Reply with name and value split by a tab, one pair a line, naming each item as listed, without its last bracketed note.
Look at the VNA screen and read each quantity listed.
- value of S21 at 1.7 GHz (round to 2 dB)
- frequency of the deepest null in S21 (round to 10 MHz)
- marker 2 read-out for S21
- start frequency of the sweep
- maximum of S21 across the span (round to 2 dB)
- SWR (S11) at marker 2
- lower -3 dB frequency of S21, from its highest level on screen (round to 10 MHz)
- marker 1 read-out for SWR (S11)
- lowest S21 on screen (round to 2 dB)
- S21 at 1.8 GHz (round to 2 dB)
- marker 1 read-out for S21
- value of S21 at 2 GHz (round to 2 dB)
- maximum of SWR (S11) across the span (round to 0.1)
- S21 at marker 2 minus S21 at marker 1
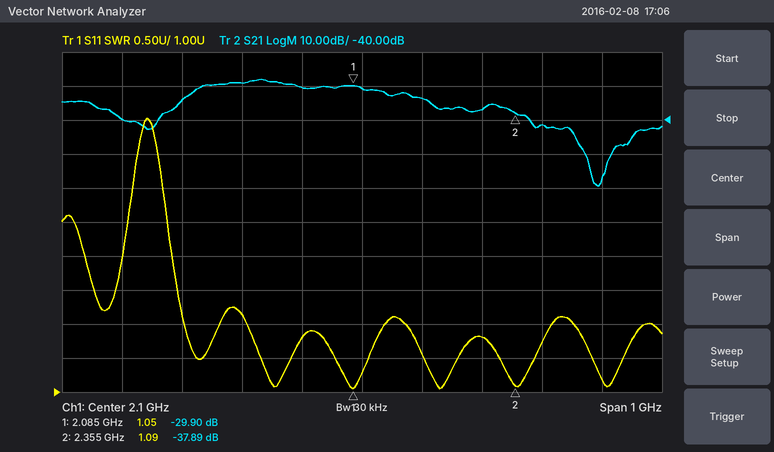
value of S21 at 1.7 GHz	-40 dB
frequency of the deepest null in S21	2.49 GHz
marker 2 read-out for S21	-37.89 dB
start frequency of the sweep	1.6 GHz
maximum of S21 across the span	-28 dB
SWR (S11) at marker 2	1.09
lower -3 dB frequency of S21, from its highest level on screen	1.82 GHz
marker 1 read-out for SWR	1.05
lowest S21 on screen	-60 dB
S21 at 1.8 GHz	-34 dB
marker 1 read-out for S21	-29.90 dB
value of S21 at 2 GHz	-30 dB
maximum of SWR (S11) across the span	5.0
S21 at marker 2 minus S21 at marker 1	-7.99 dB
